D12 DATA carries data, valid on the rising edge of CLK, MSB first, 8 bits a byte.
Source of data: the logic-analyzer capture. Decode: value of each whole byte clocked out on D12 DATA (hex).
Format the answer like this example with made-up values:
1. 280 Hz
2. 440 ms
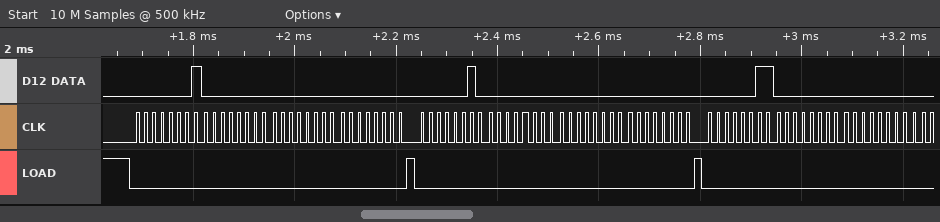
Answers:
1. 01 00 00 00 02 00 00 00 03 00 00
